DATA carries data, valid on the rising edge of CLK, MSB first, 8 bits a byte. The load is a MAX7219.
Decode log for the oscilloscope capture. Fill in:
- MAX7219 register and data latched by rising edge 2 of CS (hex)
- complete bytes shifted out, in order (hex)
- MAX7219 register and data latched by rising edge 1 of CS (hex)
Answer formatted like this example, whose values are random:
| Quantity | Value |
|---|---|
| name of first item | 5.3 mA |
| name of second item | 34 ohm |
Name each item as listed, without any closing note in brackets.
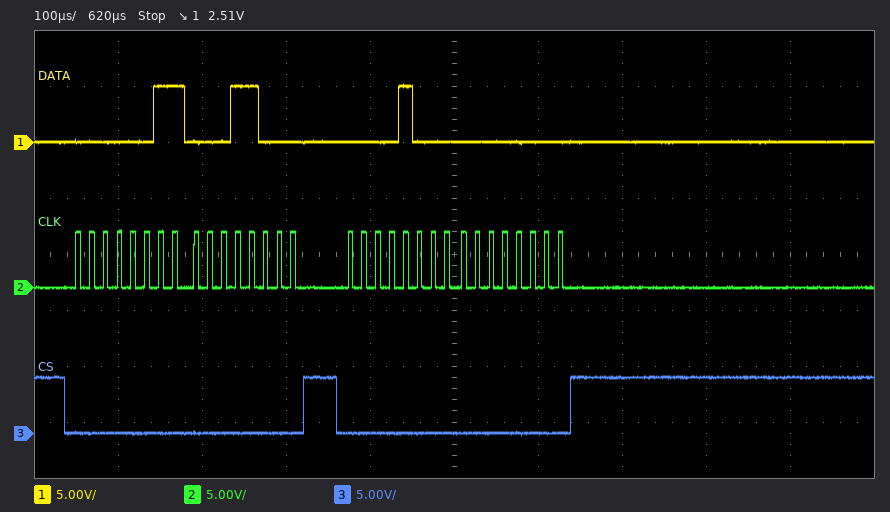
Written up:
| Quantity | Value |
|---|---|
| MAX7219 register and data latched by rising edge 2 of CS | register 0x8, data 0x00 |
| complete bytes shifted out, in order | 03 18 08 00 |
| MAX7219 register and data latched by rising edge 1 of CS | register 0x3, data 0x18 |
